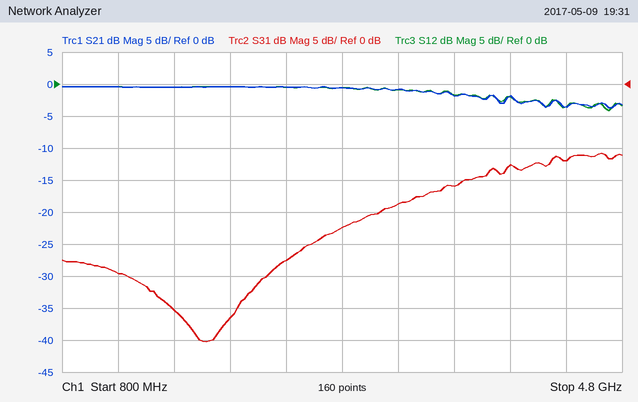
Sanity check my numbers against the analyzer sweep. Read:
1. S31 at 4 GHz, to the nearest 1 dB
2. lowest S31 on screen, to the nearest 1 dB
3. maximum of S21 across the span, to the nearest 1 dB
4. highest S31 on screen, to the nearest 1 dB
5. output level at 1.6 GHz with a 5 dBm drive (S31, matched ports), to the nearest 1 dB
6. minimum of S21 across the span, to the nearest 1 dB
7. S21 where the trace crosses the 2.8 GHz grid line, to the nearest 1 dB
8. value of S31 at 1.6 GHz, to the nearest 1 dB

-13 dB
-40 dB
0 dB
-11 dB
-30 dBm
-4 dB
-1 dB
-35 dB
